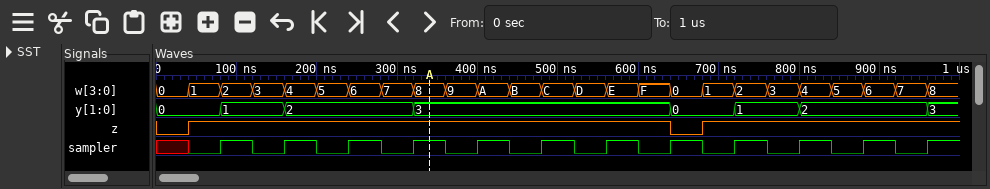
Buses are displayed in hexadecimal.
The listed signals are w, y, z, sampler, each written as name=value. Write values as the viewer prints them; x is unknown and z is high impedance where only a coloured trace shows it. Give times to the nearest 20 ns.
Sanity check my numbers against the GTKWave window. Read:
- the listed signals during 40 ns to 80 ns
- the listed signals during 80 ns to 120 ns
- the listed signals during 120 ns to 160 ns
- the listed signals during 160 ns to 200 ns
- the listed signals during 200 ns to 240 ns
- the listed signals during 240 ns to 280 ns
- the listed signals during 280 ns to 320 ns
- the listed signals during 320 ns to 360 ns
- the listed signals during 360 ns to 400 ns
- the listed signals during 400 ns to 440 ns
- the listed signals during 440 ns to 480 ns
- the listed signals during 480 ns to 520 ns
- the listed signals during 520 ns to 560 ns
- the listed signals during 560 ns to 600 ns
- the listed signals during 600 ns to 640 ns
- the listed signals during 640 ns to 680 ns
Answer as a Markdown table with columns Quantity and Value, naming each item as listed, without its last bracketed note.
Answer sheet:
| Quantity | Value |
|---|---|
| the listed signals during 40 ns to 80 ns | w=1, y=0, z=1, sampler=0 |
| the listed signals during 80 ns to 120 ns | w=2, y=1, z=1, sampler=1 |
| the listed signals during 120 ns to 160 ns | w=3, y=1, z=1, sampler=0 |
| the listed signals during 160 ns to 200 ns | w=4, y=2, z=1, sampler=1 |
| the listed signals during 200 ns to 240 ns | w=5, y=2, z=1, sampler=0 |
| the listed signals during 240 ns to 280 ns | w=6, y=2, z=1, sampler=1 |
| the listed signals during 280 ns to 320 ns | w=7, y=2, z=1, sampler=0 |
| the listed signals during 320 ns to 360 ns | w=8, y=3, z=1, sampler=1 |
| the listed signals during 360 ns to 400 ns | w=9, y=3, z=1, sampler=0 |
| the listed signals during 400 ns to 440 ns | w=A, y=3, z=1, sampler=1 |
| the listed signals during 440 ns to 480 ns | w=B, y=3, z=1, sampler=0 |
| the listed signals during 480 ns to 520 ns | w=C, y=3, z=1, sampler=1 |
| the listed signals during 520 ns to 560 ns | w=D, y=3, z=1, sampler=0 |
| the listed signals during 560 ns to 600 ns | w=E, y=3, z=1, sampler=1 |
| the listed signals during 600 ns to 640 ns | w=F, y=3, z=1, sampler=0 |
| the listed signals during 640 ns to 680 ns | w=0, y=0, z=0, sampler=1 |
